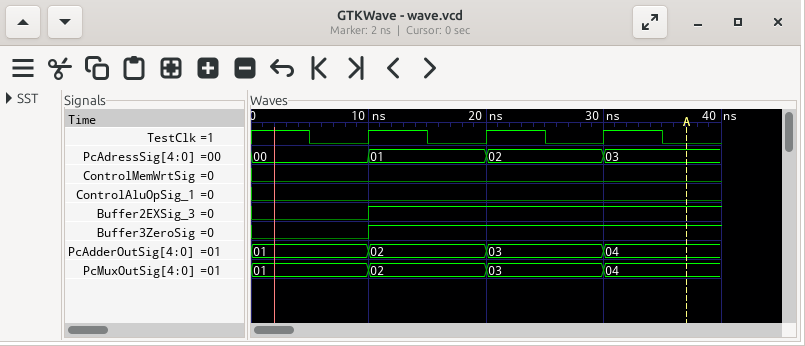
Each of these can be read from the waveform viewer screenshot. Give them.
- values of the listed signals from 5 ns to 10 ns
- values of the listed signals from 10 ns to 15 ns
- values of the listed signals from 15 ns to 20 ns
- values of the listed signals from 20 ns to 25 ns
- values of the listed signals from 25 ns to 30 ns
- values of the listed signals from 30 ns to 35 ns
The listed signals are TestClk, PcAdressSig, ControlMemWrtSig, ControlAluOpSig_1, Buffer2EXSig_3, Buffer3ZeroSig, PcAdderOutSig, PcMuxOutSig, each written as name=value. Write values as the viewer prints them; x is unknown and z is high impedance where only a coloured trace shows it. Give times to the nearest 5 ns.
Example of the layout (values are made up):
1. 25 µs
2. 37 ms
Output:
1. TestClk=0, PcAdressSig=00, ControlMemWrtSig=0, ControlAluOpSig_1=0, Buffer2EXSig_3=0, Buffer3ZeroSig=0, PcAdderOutSig=01, PcMuxOutSig=01
2. TestClk=1, PcAdressSig=01, ControlMemWrtSig=0, ControlAluOpSig_1=0, Buffer2EXSig_3=1, Buffer3ZeroSig=1, PcAdderOutSig=02, PcMuxOutSig=02
3. TestClk=0, PcAdressSig=01, ControlMemWrtSig=0, ControlAluOpSig_1=0, Buffer2EXSig_3=1, Buffer3ZeroSig=1, PcAdderOutSig=02, PcMuxOutSig=02
4. TestClk=1, PcAdressSig=02, ControlMemWrtSig=0, ControlAluOpSig_1=0, Buffer2EXSig_3=1, Buffer3ZeroSig=1, PcAdderOutSig=03, PcMuxOutSig=03
5. TestClk=0, PcAdressSig=02, ControlMemWrtSig=0, ControlAluOpSig_1=0, Buffer2EXSig_3=1, Buffer3ZeroSig=1, PcAdderOutSig=03, PcMuxOutSig=03
6. TestClk=1, PcAdressSig=03, ControlMemWrtSig=0, ControlAluOpSig_1=0, Buffer2EXSig_3=1, Buffer3ZeroSig=1, PcAdderOutSig=04, PcMuxOutSig=04
